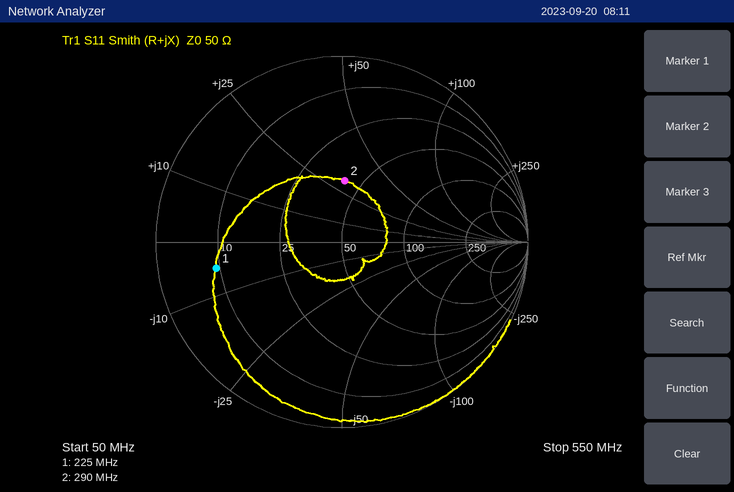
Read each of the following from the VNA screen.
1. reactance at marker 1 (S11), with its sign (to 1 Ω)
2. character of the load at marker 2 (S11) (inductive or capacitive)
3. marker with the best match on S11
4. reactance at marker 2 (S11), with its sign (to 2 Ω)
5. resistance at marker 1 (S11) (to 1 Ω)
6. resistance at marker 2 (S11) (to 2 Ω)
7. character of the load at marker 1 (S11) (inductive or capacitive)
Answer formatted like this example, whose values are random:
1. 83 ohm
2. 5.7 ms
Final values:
1. -5 Ω
2. inductive
3. marker 2
4. +30 Ω
5. 9 Ω
6. 42 Ω
7. capacitive
